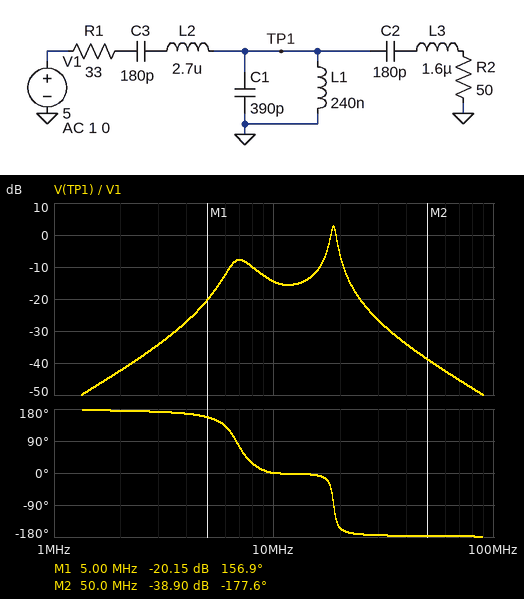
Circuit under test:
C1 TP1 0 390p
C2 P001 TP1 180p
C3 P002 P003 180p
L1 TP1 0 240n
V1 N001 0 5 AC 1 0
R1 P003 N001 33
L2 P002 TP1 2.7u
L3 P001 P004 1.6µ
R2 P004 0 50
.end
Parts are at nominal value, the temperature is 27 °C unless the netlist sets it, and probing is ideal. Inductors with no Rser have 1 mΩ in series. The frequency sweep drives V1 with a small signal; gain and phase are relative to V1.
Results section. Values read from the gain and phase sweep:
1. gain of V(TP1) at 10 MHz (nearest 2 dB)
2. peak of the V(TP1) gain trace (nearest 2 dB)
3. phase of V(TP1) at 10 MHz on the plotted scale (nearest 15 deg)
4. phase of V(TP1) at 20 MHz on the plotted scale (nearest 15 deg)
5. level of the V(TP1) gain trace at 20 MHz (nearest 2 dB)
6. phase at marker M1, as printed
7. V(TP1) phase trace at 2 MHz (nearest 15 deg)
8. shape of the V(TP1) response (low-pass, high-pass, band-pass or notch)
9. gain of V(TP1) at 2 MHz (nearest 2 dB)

-14 dB
2 dB
0 deg
-150 deg
-6 dB
156.9 deg
180 deg
band-pass
-42 dB
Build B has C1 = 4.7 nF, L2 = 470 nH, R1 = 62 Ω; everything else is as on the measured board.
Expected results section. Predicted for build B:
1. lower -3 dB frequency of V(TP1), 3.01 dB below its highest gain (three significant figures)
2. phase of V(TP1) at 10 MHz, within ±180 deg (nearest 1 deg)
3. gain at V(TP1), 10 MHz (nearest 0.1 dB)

4.50 MHz
-40 deg
-26.0 dB
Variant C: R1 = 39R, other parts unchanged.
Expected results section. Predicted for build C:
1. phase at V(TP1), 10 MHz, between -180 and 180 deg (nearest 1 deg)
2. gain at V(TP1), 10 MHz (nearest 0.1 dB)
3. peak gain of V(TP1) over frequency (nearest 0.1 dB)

3 deg
-14.8 dB
2.4 dB
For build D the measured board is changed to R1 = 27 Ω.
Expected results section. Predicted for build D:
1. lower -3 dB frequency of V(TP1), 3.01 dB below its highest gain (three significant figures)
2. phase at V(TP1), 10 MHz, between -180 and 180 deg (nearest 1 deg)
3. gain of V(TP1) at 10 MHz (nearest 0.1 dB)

18.1 MHz
-3 deg
-14.5 dB
